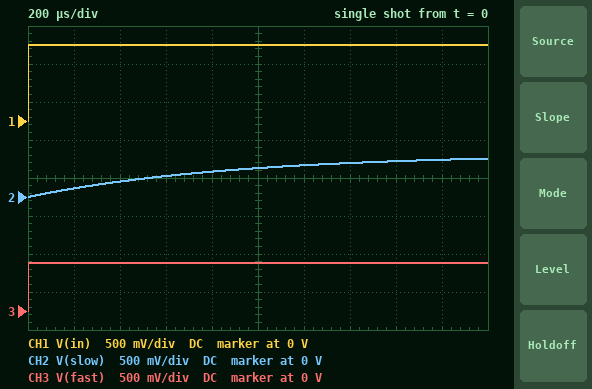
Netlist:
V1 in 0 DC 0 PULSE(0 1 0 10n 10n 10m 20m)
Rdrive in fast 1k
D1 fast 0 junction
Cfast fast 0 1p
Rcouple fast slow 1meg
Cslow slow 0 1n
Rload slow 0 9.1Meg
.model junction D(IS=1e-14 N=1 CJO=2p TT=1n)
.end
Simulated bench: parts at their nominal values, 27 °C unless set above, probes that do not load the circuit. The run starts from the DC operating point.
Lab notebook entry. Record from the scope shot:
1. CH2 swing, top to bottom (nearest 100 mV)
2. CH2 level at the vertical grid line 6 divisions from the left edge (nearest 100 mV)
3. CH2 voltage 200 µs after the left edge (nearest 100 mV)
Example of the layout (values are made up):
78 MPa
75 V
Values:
500 mV
400 mV
100 mV
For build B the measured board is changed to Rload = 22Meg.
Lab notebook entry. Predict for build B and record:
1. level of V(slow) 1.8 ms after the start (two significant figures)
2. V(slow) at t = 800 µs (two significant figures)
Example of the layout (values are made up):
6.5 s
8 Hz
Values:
510 mV
340 mV
